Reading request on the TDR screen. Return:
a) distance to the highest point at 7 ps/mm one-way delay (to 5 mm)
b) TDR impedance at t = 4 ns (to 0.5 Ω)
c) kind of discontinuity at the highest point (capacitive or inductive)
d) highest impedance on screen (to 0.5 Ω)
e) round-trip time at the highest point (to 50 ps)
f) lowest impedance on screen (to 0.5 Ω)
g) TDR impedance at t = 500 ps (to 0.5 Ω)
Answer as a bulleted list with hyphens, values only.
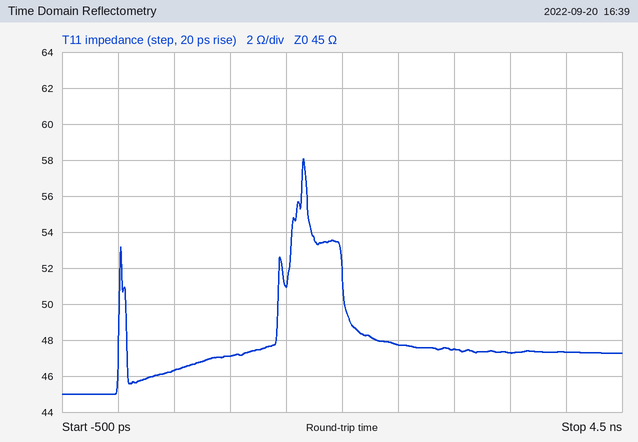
- 120 mm
- 47.5 Ω
- inductive
- 58.0 Ω
- 1.65 ns
- 45.0 Ω
- 46.5 Ω
